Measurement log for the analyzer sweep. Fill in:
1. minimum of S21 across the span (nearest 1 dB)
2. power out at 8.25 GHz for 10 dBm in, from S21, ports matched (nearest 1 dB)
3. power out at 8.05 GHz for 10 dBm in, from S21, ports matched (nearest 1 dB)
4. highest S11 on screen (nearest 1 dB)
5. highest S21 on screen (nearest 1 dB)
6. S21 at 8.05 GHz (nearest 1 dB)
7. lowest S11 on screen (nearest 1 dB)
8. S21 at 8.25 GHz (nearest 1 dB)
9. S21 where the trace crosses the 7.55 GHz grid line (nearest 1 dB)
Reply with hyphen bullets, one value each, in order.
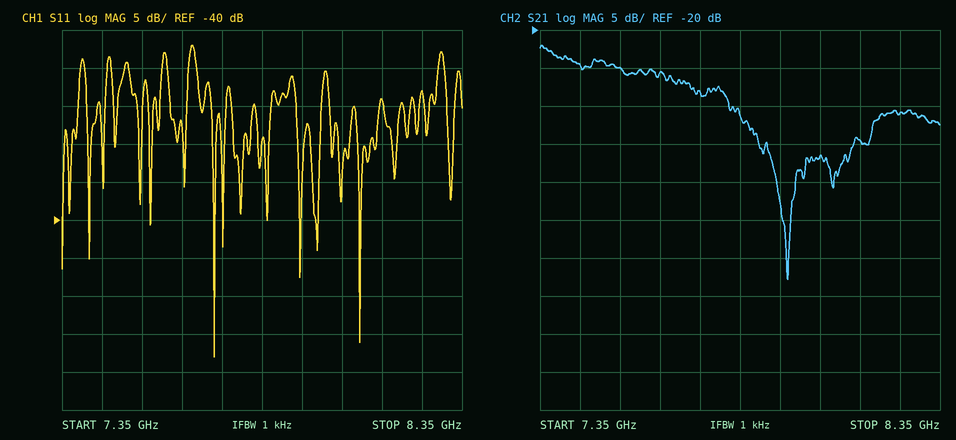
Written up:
- -53 dB
- -21 dBm
- -27 dBm
- -17 dB
- -22 dB
- -37 dB
- -58 dB
- -31 dB
- -25 dB
